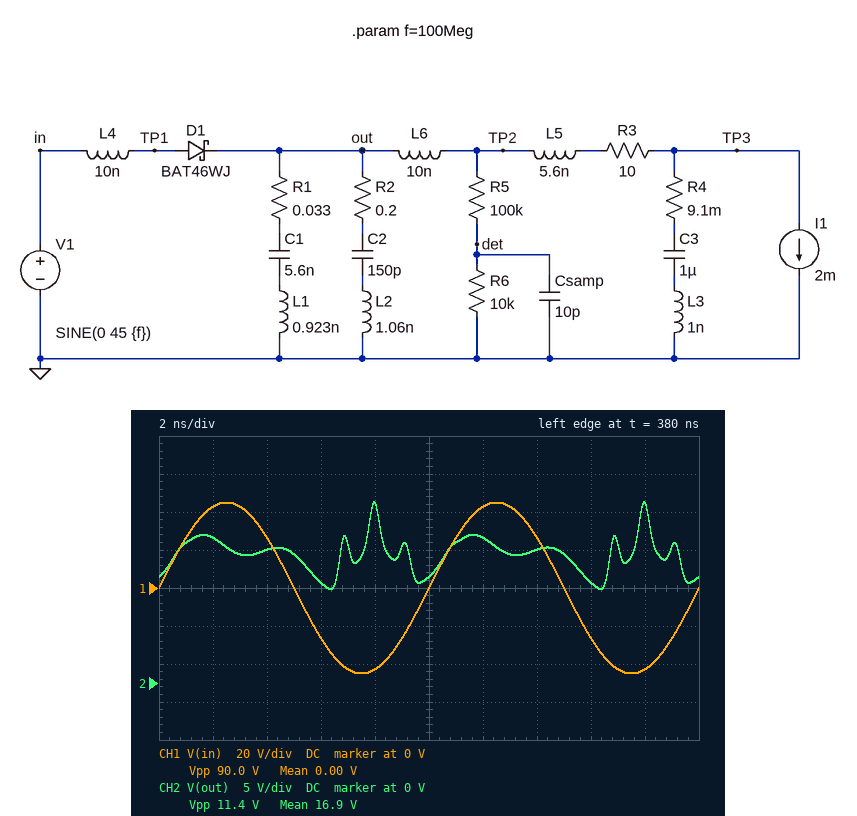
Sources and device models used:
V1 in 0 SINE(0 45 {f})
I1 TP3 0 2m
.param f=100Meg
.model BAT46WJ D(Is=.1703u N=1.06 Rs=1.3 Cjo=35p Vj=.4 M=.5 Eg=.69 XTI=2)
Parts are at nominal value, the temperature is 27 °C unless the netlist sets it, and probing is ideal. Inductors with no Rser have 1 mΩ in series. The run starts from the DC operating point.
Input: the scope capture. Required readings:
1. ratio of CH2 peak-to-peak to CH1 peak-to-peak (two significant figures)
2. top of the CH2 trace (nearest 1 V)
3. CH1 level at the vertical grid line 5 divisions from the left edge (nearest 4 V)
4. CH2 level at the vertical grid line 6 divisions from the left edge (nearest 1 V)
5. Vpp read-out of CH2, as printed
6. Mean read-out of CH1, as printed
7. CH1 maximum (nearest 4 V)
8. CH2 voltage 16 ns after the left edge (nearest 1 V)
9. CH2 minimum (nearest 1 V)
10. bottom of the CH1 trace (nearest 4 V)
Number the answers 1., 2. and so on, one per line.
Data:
1. 0.13
2. 24 V
3. 0 V
4. 19 V
5. 11.4 V
6. 0.00 V
7. 44 V
8. 13 V
9. 12 V
10. -44 V
